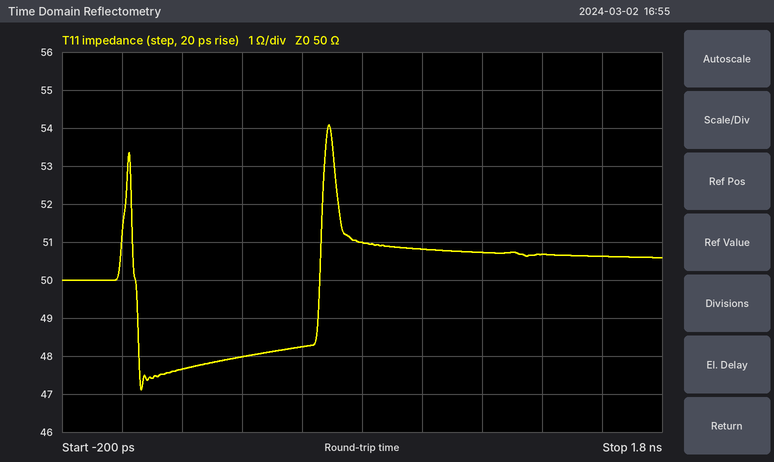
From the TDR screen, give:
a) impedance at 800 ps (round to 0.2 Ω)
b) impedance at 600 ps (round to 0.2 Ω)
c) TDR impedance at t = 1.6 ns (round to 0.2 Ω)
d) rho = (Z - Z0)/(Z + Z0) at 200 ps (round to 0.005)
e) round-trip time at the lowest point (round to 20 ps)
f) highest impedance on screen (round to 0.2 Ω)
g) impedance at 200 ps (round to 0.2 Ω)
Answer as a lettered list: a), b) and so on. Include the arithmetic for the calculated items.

a) 51.0 Ω
b) 48.2 Ω
c) 50.6 Ω
d) (47.6 − 50)/(47.6 + 50) ≈ -0.025
e) 60 ps
f) 54.0 Ω
g) 47.6 Ω
